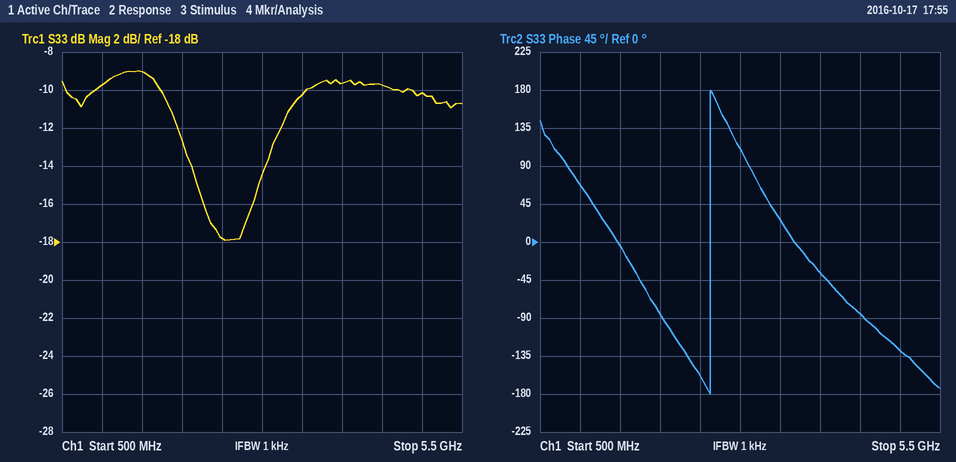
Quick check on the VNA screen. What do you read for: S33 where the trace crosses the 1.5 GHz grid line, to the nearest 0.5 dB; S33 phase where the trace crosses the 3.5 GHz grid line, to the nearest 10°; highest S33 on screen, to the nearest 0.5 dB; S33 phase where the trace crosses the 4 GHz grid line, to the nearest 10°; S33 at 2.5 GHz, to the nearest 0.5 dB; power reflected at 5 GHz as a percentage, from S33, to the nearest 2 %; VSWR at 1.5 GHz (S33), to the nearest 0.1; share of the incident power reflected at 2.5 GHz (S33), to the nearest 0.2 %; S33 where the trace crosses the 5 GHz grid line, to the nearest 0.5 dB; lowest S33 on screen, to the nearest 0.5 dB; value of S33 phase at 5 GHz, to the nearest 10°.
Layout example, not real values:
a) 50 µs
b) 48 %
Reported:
a) -9.0 dB
b) 30°
c) -9.0 dB
d) -40°
e) -18.0 dB
f) 10 %
g) 2.1
h) 1.6 %
i) -10.0 dB
j) -18.0 dB
k) -130°
